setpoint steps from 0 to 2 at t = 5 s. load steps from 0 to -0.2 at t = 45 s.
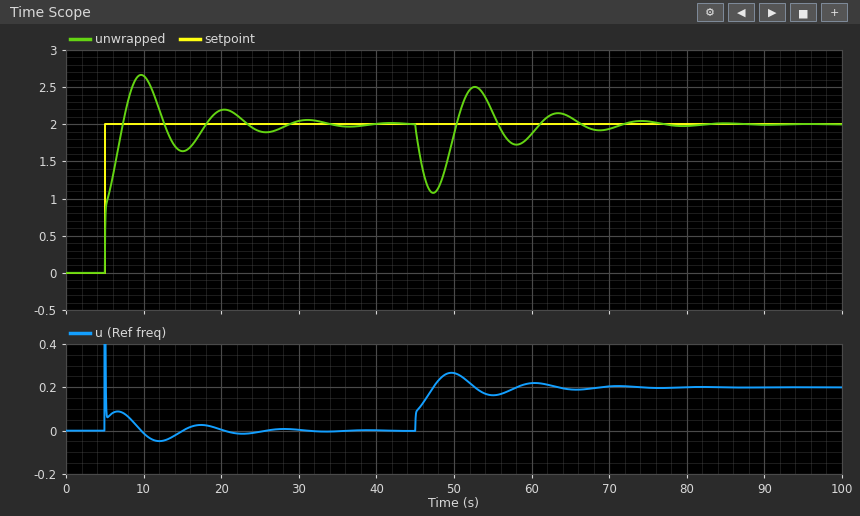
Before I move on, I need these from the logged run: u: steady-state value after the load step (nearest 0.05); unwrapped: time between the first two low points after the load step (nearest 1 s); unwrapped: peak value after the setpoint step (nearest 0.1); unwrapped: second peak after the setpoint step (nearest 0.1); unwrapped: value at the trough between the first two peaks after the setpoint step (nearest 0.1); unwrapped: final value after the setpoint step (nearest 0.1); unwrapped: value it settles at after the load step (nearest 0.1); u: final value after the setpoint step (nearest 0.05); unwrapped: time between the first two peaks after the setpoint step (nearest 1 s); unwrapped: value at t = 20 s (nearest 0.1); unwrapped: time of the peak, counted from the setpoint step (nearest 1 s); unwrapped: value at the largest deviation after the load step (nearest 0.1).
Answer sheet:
0.20
11 s
2.7
2.2
1.6
2.0
2.0
0.00
11 s
2.2
5 s
1.1
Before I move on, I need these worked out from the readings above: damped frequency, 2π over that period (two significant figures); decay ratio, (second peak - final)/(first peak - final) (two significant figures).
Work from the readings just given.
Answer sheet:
0.57 rad/s
0.29
